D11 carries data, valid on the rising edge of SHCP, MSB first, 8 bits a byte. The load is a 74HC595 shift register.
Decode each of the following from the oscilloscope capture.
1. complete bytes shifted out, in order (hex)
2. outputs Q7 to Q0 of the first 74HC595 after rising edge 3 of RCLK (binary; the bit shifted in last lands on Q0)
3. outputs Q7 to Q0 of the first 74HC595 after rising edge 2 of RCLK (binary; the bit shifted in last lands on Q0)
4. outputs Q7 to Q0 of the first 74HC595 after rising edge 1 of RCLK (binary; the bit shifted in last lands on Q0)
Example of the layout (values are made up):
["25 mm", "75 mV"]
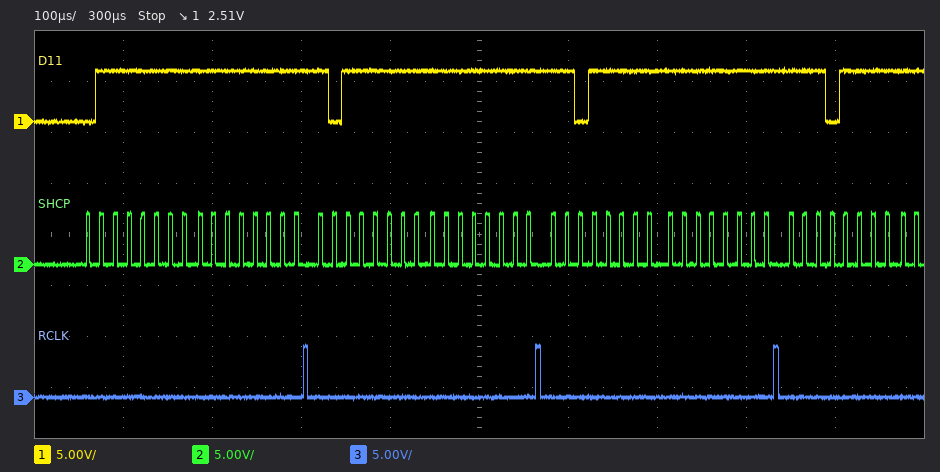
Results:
["7F FF BF FF DF FF EF", "11111111", "11111111", "11111111"]
